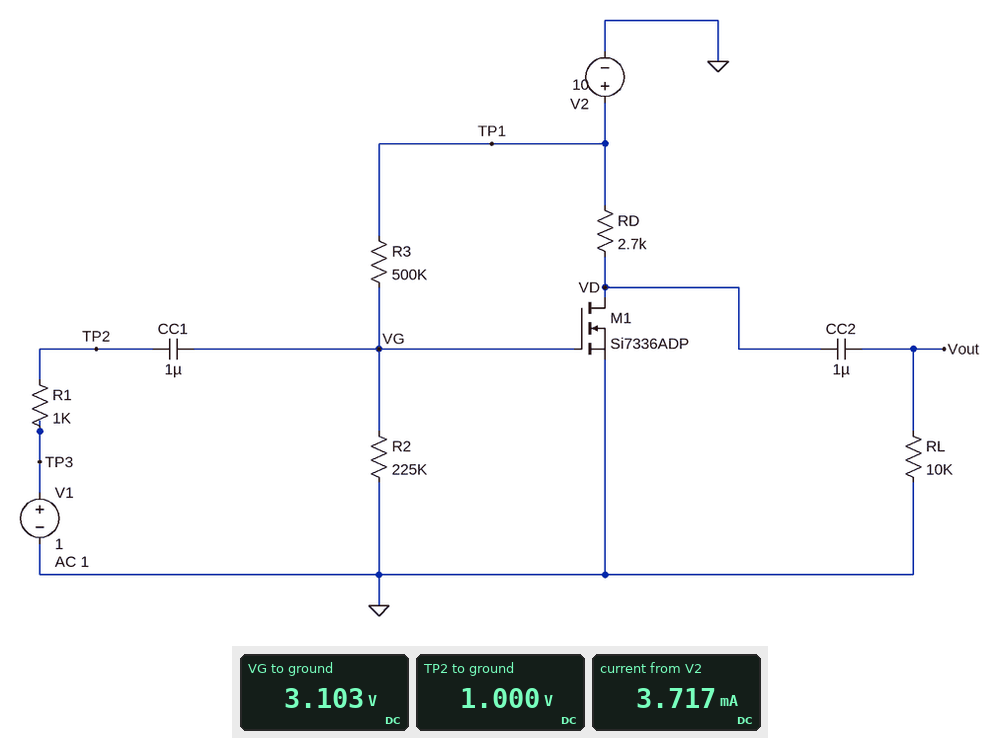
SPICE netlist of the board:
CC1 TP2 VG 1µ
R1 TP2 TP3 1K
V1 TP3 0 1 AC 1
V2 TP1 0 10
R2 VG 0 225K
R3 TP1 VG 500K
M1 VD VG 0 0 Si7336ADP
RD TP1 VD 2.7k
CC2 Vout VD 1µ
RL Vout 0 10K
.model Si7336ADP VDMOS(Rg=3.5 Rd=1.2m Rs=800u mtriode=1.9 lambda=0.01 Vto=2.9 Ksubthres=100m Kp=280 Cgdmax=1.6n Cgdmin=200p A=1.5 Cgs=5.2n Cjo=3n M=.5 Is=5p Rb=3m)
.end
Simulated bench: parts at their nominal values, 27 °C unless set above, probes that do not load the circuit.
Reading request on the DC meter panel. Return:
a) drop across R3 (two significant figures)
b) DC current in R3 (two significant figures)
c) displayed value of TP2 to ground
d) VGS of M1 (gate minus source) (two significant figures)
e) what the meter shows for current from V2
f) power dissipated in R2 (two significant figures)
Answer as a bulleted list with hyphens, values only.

- 6.9 V
- 14 µA
- 1.000 V
- 3.1 V
- 3.717 mA
- 43 µW
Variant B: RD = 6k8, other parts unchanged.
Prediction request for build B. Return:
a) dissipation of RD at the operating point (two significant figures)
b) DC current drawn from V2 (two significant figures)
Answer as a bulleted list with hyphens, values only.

- 15 mW
- 1.5 mA
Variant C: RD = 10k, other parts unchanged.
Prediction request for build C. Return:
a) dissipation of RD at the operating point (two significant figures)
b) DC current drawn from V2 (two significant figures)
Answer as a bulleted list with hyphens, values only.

- 10 mW
- 1.0 mA
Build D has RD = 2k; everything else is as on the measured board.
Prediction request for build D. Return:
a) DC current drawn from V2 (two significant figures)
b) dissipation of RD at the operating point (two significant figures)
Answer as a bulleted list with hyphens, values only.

- 5.0 mA
- 50 mW
